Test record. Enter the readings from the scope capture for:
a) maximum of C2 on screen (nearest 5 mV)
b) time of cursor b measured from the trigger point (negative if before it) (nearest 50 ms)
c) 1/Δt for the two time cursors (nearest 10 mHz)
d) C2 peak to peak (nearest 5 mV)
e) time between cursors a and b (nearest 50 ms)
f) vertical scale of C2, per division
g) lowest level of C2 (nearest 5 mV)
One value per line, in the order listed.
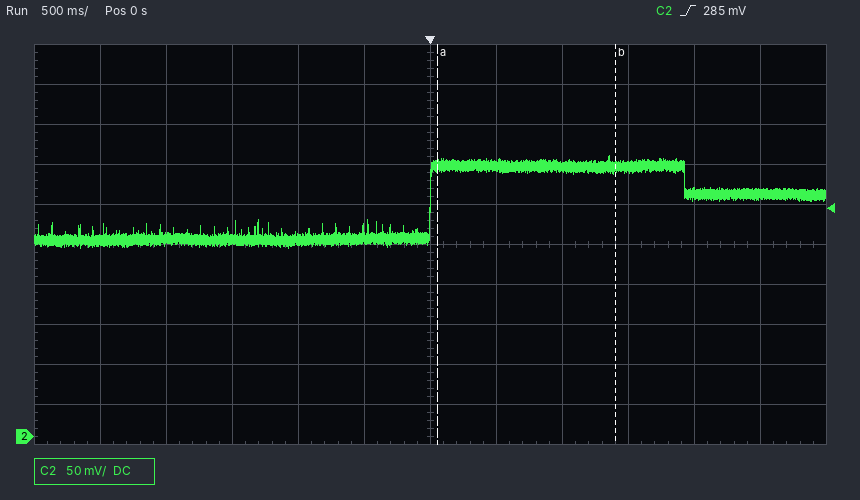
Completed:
350 mV
+1.40 s
740 mHz
115 mV
1.35 s
50 mV
235 mV
